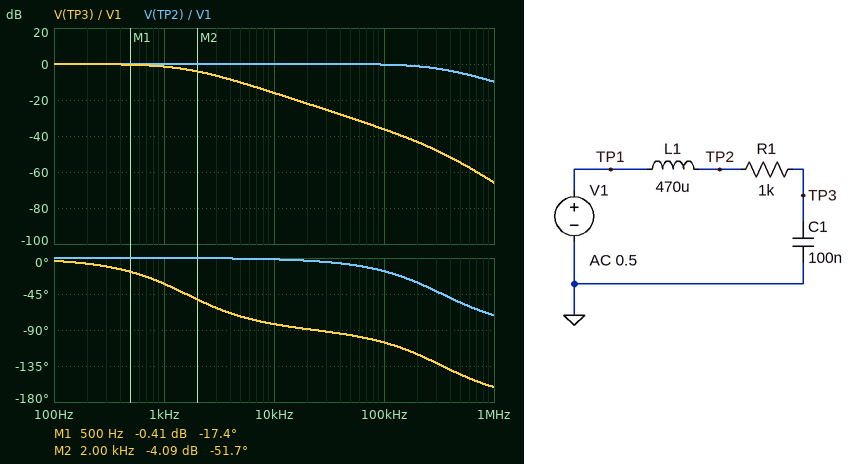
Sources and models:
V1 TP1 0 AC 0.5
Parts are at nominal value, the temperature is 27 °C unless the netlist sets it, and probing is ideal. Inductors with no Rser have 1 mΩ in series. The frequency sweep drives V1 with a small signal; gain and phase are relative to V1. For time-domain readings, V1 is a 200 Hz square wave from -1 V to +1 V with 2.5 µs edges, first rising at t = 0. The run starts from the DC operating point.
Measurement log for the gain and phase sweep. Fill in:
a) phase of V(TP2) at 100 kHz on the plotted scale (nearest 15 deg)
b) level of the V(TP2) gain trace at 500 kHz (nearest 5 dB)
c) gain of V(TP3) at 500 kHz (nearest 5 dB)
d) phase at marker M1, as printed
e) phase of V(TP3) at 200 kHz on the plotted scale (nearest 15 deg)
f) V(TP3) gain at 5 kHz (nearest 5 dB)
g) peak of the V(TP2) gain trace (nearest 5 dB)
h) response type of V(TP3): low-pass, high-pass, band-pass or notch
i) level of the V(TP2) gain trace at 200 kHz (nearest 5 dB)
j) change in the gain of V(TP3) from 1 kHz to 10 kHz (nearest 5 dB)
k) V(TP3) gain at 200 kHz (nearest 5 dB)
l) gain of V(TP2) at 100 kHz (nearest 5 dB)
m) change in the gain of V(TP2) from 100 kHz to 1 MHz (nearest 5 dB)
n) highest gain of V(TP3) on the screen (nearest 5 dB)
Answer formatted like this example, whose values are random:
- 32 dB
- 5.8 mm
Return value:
- -15 deg
- -5 dB
- -55 dB
- -17.4 deg
- -120 deg
- -10 dB
- 0 dB
- low-pass
- 0 dB
- -15 dB
- -45 dB
- 0 dB
- -10 dB
- 0 dB
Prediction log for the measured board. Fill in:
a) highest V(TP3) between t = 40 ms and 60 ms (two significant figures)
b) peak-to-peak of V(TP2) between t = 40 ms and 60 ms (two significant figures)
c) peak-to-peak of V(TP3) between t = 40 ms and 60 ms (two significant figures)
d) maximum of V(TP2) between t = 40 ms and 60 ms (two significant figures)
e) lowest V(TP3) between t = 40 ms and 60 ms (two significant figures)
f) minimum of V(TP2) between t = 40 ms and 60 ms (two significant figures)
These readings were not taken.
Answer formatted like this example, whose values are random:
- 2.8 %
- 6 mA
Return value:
- 1.0 V
- 2.0 V
- 2.0 V
- 1.0 V
- -1.0 V
- -1.0 V
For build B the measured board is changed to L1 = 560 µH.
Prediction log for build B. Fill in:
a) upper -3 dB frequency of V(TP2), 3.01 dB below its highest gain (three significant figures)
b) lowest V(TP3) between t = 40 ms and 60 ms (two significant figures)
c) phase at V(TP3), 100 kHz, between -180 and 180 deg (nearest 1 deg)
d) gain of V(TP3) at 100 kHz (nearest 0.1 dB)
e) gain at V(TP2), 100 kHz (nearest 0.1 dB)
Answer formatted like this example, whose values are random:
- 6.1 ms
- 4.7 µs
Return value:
- 283 kHz
- -1.0 V
- -109 deg
- -36.4 dB
- -0.5 dB
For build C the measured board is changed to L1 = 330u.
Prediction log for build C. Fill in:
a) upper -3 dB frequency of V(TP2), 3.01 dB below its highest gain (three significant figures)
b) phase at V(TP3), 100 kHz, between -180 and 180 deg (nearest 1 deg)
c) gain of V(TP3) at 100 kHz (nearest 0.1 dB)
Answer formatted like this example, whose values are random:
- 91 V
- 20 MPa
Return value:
- 481 kHz
- -101 deg
- -36.1 dB
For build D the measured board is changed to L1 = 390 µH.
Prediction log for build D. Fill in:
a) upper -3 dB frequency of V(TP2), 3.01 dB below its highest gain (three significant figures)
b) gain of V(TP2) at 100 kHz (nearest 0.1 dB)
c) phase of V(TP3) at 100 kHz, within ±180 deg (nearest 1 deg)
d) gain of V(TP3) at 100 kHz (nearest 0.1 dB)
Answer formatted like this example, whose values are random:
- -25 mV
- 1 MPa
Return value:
- 407 kHz
- -0.2 dB
- -103 deg
- -36.2 dB
